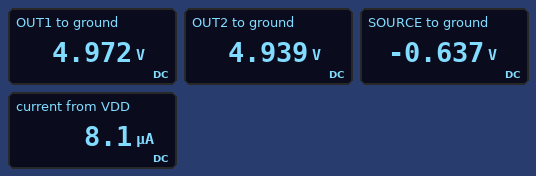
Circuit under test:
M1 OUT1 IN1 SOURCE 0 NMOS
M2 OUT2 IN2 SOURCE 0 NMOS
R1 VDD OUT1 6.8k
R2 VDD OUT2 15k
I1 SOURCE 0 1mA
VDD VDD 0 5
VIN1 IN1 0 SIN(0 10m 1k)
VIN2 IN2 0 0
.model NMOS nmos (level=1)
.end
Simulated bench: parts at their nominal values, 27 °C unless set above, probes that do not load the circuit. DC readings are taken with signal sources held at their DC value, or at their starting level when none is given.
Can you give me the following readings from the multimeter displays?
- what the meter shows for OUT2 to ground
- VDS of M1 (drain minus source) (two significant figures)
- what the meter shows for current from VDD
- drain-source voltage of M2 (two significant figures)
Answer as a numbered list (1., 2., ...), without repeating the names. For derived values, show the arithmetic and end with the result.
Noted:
1. 4.939 V
2. 4.972 V - (-637 mV) = 5.6 V
3. 8.1 µA
4. 4.939 V - (-637 mV) = 5.6 V
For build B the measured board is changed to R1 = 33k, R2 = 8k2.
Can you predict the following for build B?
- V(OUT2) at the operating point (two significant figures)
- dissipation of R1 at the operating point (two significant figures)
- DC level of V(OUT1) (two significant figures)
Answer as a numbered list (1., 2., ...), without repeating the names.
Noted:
1. 5.0 V
2. 540 nW
3. 4.9 V
